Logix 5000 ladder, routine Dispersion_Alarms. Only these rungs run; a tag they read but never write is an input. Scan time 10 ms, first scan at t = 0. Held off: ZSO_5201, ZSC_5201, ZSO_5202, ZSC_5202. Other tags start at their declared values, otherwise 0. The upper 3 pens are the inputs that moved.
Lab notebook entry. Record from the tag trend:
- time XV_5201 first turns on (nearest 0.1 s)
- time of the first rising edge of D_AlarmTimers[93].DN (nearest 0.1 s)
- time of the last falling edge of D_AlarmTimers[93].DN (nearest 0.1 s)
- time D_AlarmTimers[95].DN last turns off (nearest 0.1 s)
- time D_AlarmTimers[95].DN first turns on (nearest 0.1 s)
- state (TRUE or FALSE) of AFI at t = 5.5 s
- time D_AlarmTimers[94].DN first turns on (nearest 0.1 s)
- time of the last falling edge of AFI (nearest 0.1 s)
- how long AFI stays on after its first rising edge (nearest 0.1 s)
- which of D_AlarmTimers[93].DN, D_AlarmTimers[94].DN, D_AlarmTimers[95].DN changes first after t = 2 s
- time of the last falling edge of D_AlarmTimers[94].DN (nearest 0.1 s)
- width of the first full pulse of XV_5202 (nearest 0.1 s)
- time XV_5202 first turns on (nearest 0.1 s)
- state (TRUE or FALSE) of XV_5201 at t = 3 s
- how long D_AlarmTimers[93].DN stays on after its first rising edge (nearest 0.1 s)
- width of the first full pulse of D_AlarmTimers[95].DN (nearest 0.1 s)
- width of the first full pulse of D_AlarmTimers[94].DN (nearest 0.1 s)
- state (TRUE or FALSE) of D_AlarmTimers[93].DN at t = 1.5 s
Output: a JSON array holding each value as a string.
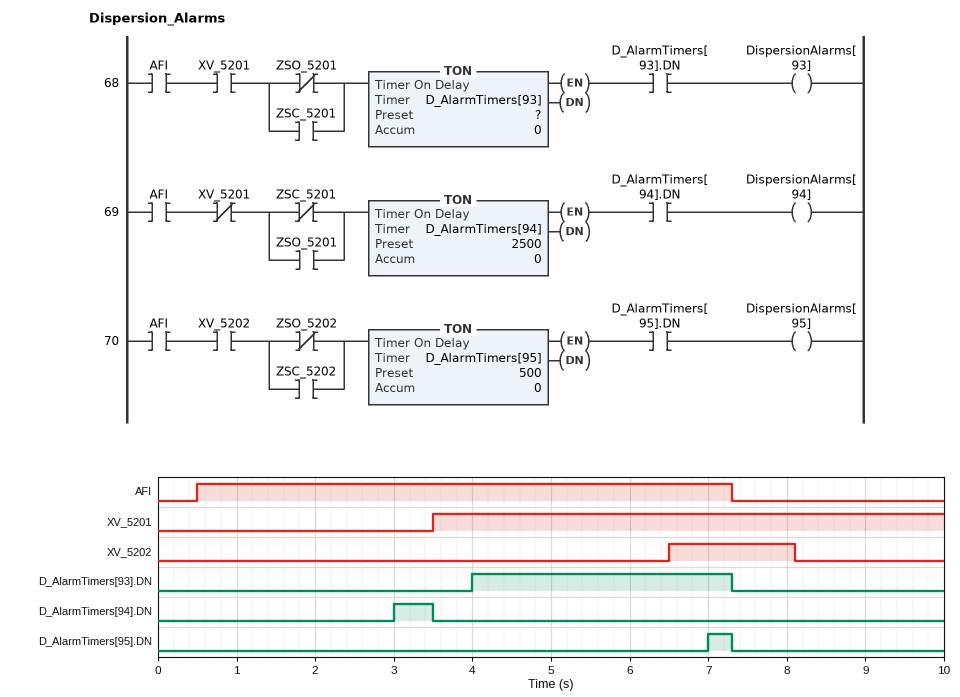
["3.5 s", "4.0 s", "7.3 s", "7.3 s", "7.0 s", "TRUE", "3.0 s", "7.3 s", "6.8 s", "D_AlarmTimers[94].DN", "3.5 s", "1.6 s", "6.5 s", "FALSE", "3.3 s", "0.3 s", "0.5 s", "FALSE"]
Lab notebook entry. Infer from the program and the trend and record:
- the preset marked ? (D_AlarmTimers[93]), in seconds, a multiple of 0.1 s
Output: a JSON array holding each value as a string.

["0.5 s"]
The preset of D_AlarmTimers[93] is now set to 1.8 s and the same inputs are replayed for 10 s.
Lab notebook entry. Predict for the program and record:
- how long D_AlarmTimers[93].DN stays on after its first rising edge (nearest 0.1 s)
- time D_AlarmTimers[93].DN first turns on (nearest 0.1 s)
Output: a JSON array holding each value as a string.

["2.0 s", "5.3 s"]
